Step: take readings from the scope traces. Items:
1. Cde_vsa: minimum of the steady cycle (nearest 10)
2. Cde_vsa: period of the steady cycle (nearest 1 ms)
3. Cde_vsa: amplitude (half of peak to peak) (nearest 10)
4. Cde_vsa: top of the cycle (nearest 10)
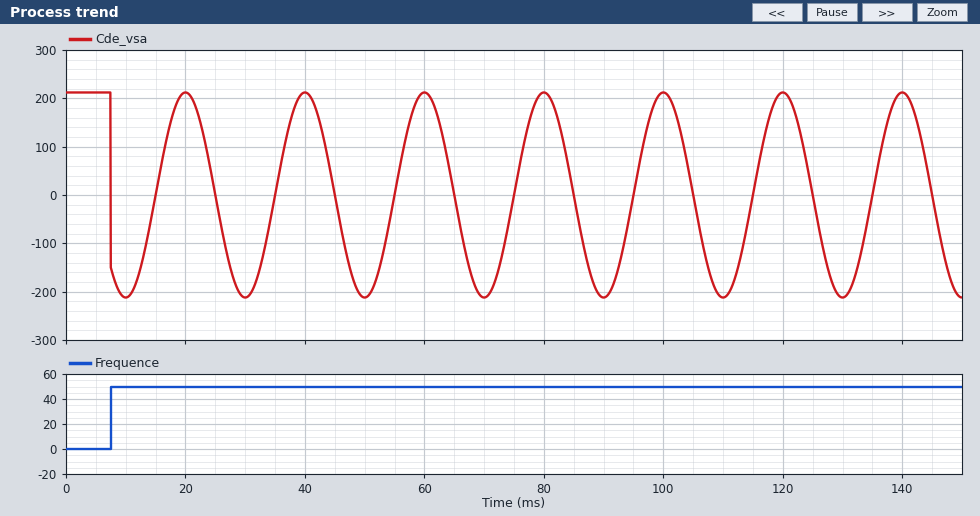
-210
20 ms
210
210
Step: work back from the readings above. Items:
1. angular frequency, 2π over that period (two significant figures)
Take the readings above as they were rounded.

0.31 rad/ms
